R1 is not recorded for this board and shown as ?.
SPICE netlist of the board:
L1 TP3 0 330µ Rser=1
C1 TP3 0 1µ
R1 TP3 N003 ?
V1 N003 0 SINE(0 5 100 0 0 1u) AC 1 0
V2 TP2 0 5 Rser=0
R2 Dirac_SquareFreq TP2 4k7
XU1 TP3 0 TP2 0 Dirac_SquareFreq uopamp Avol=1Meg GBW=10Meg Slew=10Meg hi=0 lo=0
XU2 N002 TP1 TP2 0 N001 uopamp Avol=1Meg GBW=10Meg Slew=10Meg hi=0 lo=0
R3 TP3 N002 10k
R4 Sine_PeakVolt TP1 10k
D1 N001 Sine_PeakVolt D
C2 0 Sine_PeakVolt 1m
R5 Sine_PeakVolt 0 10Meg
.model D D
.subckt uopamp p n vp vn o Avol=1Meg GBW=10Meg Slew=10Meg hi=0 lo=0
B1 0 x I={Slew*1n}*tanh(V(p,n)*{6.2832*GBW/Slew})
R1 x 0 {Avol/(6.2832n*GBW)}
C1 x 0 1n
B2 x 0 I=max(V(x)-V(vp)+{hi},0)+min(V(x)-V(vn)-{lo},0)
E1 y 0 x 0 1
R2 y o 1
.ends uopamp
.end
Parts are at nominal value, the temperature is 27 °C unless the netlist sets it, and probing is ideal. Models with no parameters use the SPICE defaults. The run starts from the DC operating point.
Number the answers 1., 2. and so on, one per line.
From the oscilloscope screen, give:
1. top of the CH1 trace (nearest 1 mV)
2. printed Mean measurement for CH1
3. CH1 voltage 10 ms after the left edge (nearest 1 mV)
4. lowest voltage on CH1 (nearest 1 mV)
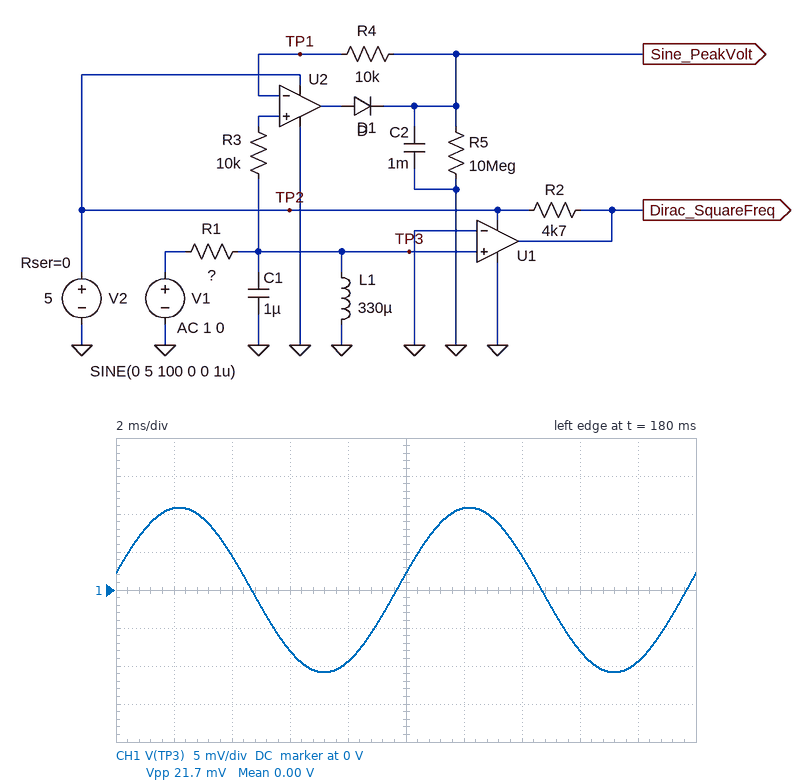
1. 11 mV
2. 0.00 V
3. 2 mV
4. -11 mV
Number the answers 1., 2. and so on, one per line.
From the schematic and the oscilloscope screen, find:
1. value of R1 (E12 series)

1. 470 Ω
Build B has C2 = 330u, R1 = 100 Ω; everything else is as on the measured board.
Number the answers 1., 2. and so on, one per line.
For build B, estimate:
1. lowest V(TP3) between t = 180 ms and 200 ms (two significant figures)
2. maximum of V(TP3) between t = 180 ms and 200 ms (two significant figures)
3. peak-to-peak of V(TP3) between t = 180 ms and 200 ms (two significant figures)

1. -51 mV
2. 51 mV
3. 100 mV
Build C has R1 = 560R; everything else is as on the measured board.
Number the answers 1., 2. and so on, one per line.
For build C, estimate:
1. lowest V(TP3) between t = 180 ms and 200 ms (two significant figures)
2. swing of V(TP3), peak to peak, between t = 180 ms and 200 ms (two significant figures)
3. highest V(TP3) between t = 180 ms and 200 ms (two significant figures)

1. -9.1 mV
2. 18 mV
3. 9.1 mV
